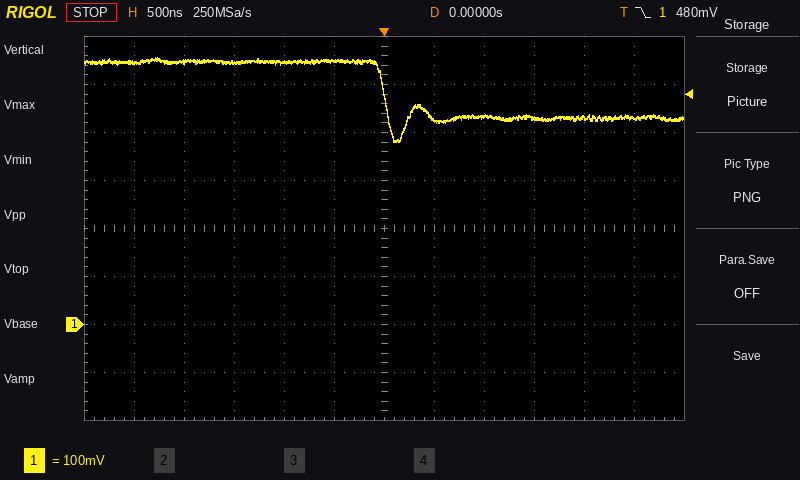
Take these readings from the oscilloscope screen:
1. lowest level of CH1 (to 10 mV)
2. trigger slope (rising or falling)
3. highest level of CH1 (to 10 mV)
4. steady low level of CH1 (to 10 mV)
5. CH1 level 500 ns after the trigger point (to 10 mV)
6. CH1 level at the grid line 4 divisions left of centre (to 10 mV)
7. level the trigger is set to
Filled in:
380 mV
falling
560 mV
430 mV
430 mV
550 mV
480 mV
